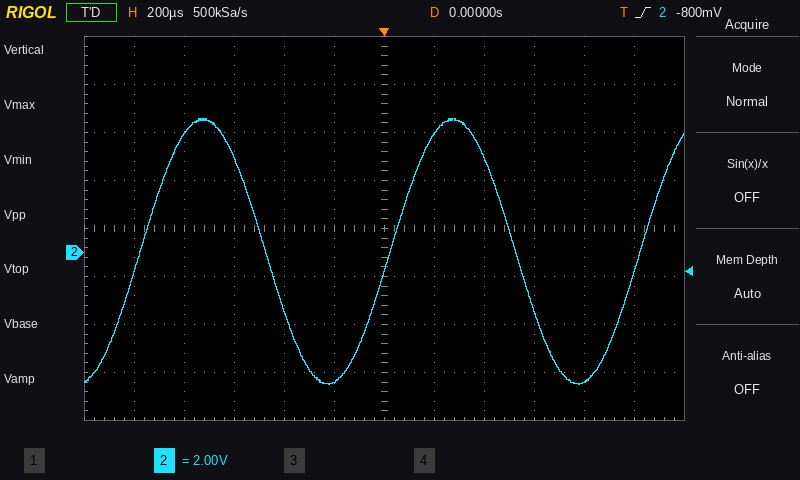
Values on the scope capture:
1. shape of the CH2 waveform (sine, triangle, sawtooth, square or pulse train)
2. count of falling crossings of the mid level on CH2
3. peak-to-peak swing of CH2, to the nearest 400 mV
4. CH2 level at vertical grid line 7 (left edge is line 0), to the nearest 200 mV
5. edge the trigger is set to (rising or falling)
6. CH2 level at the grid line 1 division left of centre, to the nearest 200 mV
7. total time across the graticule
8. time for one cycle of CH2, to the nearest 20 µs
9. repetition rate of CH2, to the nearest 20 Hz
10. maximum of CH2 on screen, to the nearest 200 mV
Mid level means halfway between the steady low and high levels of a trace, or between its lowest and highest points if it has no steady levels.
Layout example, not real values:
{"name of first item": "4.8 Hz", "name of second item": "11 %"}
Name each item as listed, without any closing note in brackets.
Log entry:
{"shape of the CH2 waveform": "sine", "count of falling crossings of the mid level on CH2": "2", "peak-to-peak swing of CH2, to the nearest 400 mV": "11.2 V", "CH2 level at vertical grid line 7 (left edge is line 0), to the nearest 200 mV": "5.0 V", "edge the trigger is set to": "rising", "CH2 level at the grid line 1 division left of centre, to the nearest 200 mV": "-5.4 V", "total time across the graticule": "2.4 ms", "time for one cycle of CH2, to the nearest 20 µs": "1.00 ms", "repetition rate of CH2, to the nearest 20 Hz": "1.00 kHz", "maximum of CH2 on screen, to the nearest 200 mV": "5.6 V"}
